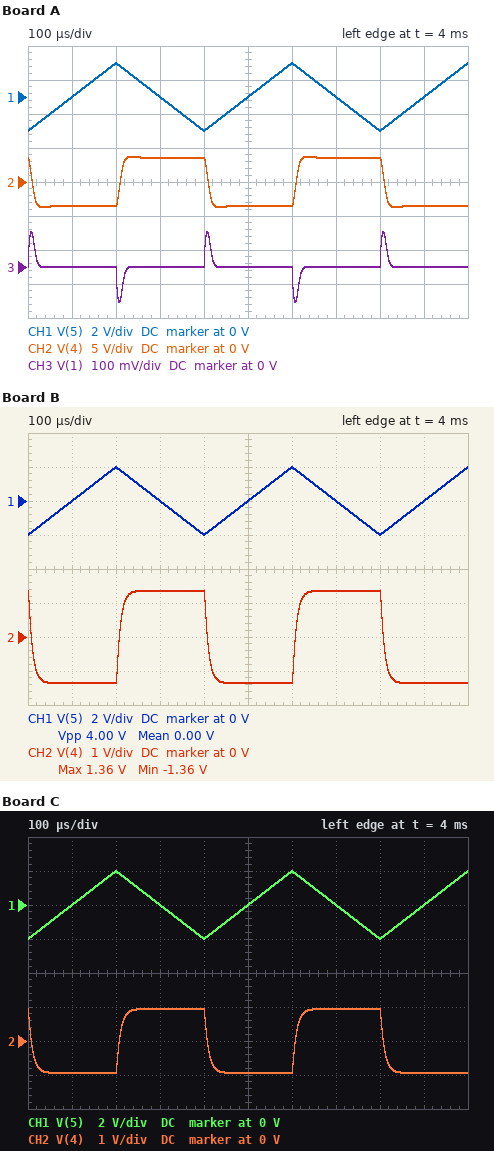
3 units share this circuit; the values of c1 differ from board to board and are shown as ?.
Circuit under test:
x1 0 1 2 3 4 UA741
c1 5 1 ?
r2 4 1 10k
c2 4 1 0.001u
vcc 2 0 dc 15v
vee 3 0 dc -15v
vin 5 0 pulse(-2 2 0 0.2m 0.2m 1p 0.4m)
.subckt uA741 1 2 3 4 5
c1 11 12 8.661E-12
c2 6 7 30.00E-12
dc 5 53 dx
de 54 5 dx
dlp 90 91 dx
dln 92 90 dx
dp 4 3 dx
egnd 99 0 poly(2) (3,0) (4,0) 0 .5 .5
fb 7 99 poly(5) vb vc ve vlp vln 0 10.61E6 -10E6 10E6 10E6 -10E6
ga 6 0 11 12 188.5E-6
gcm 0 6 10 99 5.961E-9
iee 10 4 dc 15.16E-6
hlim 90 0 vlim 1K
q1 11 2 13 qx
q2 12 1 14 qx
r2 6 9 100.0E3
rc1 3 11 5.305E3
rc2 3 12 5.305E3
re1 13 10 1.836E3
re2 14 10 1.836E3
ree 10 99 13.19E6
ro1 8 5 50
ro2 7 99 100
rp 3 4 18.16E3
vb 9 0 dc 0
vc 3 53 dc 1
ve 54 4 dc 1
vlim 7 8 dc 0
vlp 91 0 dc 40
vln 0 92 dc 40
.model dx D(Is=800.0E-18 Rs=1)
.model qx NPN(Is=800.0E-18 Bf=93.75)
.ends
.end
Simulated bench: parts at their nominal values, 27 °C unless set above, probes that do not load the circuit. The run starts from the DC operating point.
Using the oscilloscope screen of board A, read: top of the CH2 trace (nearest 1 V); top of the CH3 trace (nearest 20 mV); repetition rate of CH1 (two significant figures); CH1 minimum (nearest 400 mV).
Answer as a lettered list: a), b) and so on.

a) 4 V
b) 100 mV
c) 2.5 kHz
d) -2.0 V
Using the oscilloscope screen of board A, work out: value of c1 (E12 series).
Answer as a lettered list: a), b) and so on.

a) 18 nF
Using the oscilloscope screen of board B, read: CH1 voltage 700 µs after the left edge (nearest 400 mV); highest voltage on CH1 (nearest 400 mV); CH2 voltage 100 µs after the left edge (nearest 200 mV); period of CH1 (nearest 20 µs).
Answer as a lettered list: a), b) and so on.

a) 0 V
b) 2.0 V
c) -1.4 V
d) 400 µs
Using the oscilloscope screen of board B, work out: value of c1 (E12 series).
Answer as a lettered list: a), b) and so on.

a) 6.8 nF
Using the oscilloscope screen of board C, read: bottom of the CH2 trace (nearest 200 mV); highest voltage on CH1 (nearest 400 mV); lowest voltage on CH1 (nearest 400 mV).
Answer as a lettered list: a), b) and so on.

a) -1.0 V
b) 2.0 V
c) -2.0 V
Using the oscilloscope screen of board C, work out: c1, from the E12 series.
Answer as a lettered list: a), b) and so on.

a) 4.7 nF
